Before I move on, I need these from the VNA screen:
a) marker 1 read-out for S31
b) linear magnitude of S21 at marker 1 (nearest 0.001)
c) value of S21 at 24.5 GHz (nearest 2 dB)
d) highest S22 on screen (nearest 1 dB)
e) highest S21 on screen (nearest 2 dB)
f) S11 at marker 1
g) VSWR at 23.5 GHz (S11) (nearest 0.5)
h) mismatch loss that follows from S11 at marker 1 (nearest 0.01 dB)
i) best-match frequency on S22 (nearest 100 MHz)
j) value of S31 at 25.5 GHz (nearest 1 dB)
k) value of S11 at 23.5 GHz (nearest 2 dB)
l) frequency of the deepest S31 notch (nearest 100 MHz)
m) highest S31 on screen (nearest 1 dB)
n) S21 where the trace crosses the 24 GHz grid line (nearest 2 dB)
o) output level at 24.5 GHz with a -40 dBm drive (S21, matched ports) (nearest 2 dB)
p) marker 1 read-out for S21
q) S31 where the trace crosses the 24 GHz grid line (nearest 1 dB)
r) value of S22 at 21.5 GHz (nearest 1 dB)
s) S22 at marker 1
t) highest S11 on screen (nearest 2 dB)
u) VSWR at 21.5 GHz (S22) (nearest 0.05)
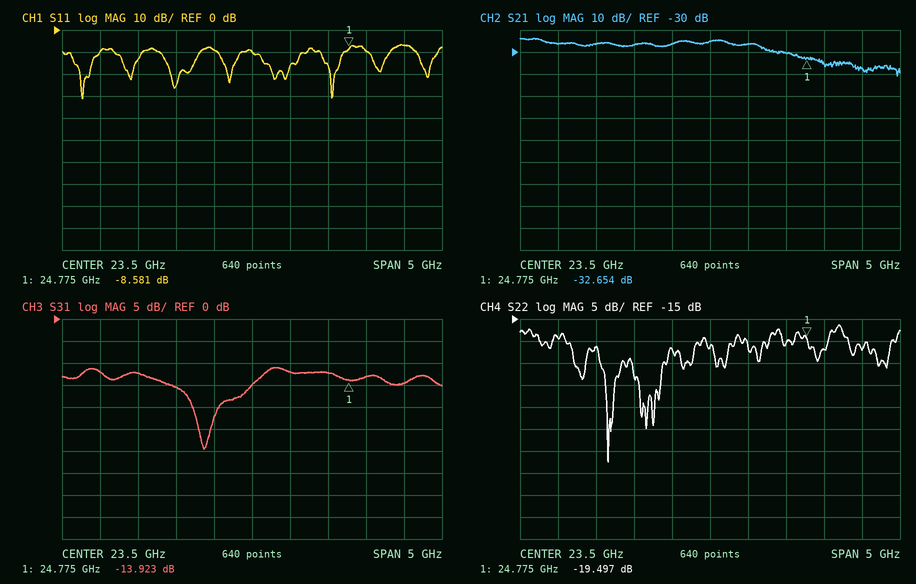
-13.923 dB
0.023
-30 dB
-16 dB
-24 dB
-8.581 dB
2.0
0.65 dB
22.2 GHz
-15 dB
-10 dB
22.9 GHz
-11 dB
-26 dB
-70 dBm
-32.654 dB
-12 dB
-19 dB
-19.497 dB
-6 dB
1.25
